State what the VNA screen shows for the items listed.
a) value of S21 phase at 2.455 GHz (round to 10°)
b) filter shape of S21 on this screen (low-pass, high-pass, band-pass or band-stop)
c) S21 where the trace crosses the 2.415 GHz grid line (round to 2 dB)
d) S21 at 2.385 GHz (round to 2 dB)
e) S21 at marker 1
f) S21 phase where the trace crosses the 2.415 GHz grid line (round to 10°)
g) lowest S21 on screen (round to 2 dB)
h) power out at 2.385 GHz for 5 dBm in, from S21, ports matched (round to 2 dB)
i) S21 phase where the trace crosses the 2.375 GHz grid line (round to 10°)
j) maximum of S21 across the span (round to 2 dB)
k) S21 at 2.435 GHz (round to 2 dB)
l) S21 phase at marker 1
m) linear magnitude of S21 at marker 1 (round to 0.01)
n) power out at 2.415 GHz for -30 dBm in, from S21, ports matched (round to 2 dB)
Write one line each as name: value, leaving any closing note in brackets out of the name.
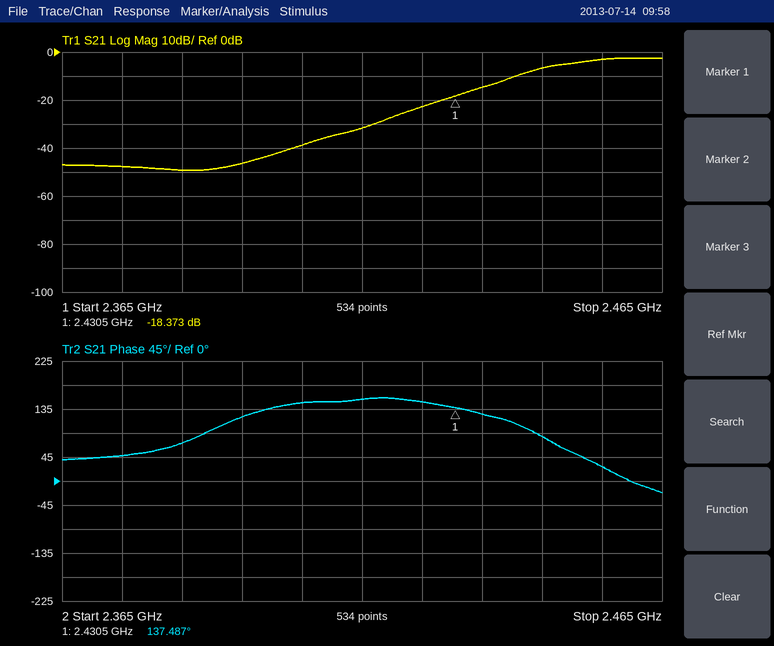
value of S21 phase at 2.455 GHz: 30°
filter shape of S21 on this screen: high-pass
S21 where the trace crosses the 2.415 GHz grid line: -32 dB
S21 at 2.385 GHz: -50 dB
S21 at marker 1: -18.373 dB
S21 phase where the trace crosses the 2.415 GHz grid line: 150°
lowest S21 on screen: -50 dB
power out at 2.385 GHz for 5 dBm in, from S21, ports matched: -44 dBm
S21 phase where the trace crosses the 2.375 GHz grid line: 50°
maximum of S21 across the span: -2 dB
S21 at 2.435 GHz: -14 dB
S21 phase at marker 1: 137.487°
linear magnitude of S21 at marker 1: 0.12
power out at 2.415 GHz for -30 dBm in, from S21, ports matched: -62 dBm
